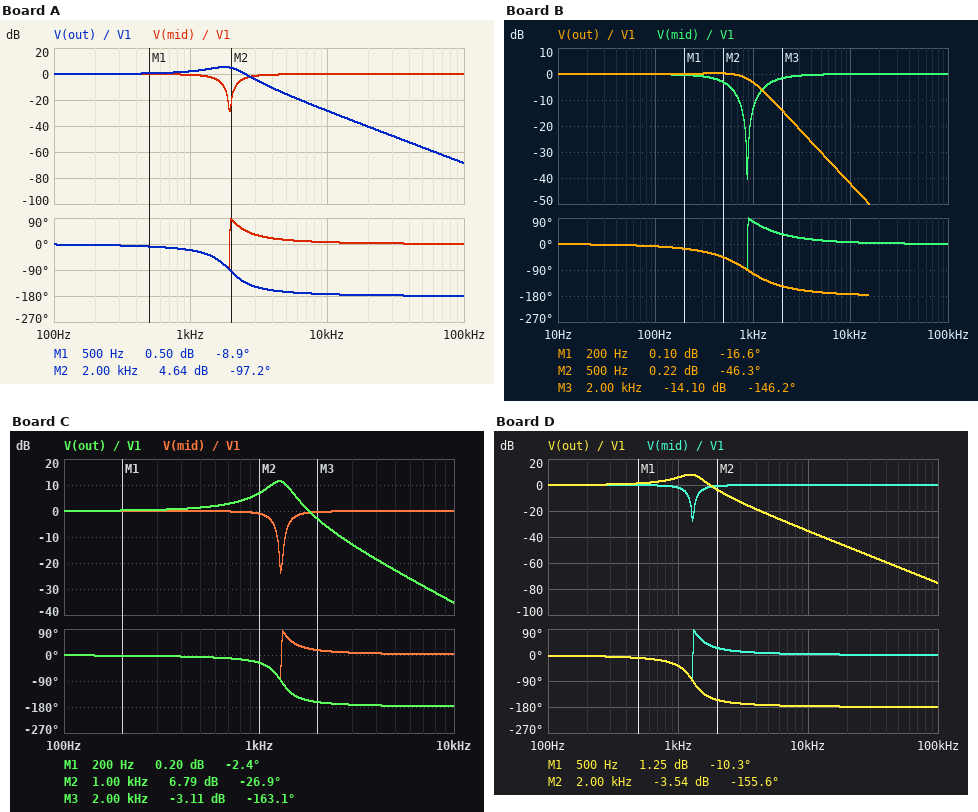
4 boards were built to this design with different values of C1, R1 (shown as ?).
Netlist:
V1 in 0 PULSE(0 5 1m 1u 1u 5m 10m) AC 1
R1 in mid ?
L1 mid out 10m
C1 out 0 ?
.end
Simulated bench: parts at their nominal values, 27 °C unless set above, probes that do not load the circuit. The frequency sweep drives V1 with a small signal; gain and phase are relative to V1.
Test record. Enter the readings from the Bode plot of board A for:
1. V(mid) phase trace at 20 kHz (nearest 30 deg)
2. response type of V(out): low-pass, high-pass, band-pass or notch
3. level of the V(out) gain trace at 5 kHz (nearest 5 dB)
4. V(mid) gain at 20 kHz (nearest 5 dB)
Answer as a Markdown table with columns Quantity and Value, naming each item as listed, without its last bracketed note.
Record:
| Quantity | Value |
|---|---|
| V(mid) phase trace at 20 kHz | 0 deg |
| response type of V(out): low-pass, high-pass, band-pass or notch | low-pass |
| level of the V(out) gain trace at 5 kHz | -15 dB |
| V(mid) gain at 20 kHz | 0 dB |
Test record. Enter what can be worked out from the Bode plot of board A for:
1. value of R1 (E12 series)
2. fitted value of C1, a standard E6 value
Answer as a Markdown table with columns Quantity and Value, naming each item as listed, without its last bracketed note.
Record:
| Quantity | Value |
|---|---|
| value of R1 | 68 Ω |
| fitted value of C1, a standard E6 value | 680 nF |
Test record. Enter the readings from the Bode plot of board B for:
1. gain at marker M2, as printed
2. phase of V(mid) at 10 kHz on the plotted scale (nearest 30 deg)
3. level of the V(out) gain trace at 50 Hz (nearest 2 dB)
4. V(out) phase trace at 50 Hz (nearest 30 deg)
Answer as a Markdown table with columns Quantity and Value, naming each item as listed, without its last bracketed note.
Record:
| Quantity | Value |
|---|---|
| gain at marker M2, as printed | 0.22 dB |
| phase of V(mid) at 10 kHz on the plotted scale | 0 deg |
| level of the V(out) gain trace at 50 Hz | 0 dB |
| V(out) phase trace at 50 Hz | 0 deg |
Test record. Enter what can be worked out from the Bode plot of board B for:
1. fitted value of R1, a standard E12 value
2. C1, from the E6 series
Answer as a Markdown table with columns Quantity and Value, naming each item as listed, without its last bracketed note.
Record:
| Quantity | Value |
|---|---|
| fitted value of R1, a standard E12 value | 68 Ω |
| C1, from the E6 series | 3.3 µF |
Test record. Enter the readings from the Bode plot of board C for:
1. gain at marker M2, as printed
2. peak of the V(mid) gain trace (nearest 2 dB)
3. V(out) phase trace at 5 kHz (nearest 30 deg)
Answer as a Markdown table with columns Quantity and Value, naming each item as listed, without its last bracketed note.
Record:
| Quantity | Value |
|---|---|
| gain at marker M2, as printed | 6.79 dB |
| peak of the V(mid) gain trace | 0 dB |
| V(out) phase trace at 5 kHz | -180 deg |
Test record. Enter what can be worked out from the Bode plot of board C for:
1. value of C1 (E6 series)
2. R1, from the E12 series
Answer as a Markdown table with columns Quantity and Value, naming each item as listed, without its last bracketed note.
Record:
| Quantity | Value |
|---|---|
| value of C1 | 1.5 µF |
| R1, from the E12 series | 22 Ω |
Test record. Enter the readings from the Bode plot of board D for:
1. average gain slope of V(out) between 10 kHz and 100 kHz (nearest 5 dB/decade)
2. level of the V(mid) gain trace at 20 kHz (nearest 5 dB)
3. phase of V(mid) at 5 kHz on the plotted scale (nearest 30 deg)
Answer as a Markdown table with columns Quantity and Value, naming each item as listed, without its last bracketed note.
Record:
| Quantity | Value |
|---|---|
| average gain slope of V(out) between 10 kHz and 100 kHz | -40 dB/decade |
| level of the V(mid) gain trace at 20 kHz | 0 dB |
| phase of V(mid) at 5 kHz on the plotted scale | 0 deg |
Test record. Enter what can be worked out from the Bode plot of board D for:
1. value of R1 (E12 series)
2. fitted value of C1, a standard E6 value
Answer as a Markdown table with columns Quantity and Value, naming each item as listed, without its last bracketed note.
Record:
| Quantity | Value |
|---|---|
| value of R1 | 33 Ω |
| fitted value of C1, a standard E6 value | 1.5 µF |
